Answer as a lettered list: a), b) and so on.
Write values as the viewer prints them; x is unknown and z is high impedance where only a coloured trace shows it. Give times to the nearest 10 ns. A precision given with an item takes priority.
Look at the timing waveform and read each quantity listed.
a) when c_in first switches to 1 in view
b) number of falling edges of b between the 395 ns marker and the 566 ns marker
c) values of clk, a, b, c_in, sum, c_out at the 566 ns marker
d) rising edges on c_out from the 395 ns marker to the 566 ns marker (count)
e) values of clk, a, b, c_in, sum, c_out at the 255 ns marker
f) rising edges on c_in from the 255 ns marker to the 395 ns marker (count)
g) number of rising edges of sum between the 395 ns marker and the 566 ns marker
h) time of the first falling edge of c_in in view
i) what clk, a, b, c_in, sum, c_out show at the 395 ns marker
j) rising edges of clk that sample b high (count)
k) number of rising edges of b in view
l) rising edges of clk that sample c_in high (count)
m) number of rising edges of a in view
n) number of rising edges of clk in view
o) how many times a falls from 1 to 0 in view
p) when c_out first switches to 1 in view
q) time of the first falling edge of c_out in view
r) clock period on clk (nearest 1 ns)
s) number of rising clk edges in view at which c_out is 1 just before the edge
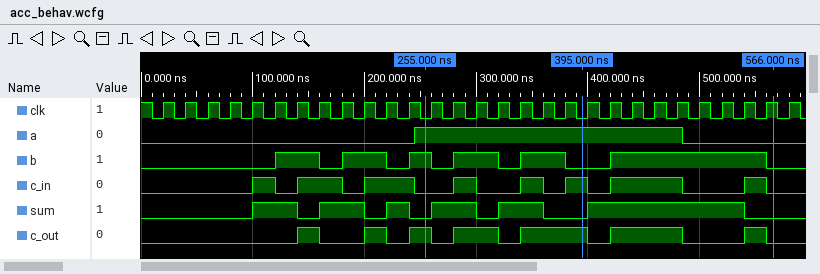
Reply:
a) 100 ns
b) 1
c) clk=1, a=0, b=0, c_in=0, sum=0, c_out=0
d) 2
e) clk=0, a=1, b=1, c_in=0, sum=0, c_out=1
f) 3
g) 1
h) 120 ns
i) clk=0, a=1, b=0, c_in=1, sum=0, c_out=1
j) 16
k) 6
l) 12
m) 1
n) 29
o) 1
p) 140 ns
q) 160 ns
r) 20 ns
s) 12
